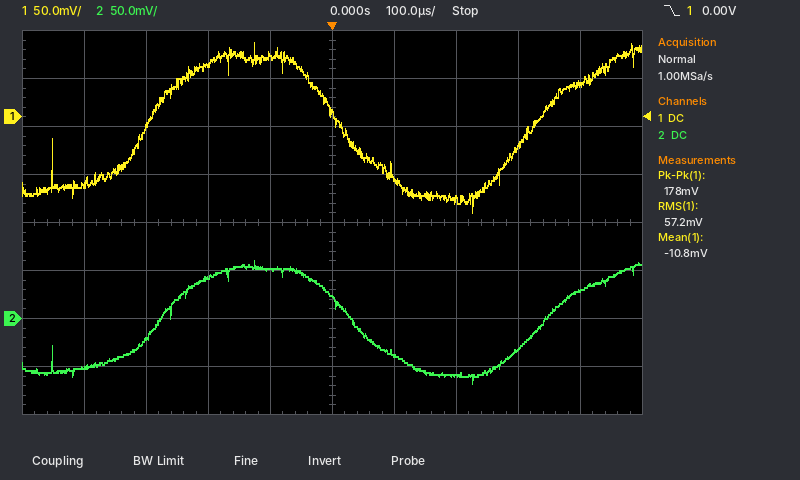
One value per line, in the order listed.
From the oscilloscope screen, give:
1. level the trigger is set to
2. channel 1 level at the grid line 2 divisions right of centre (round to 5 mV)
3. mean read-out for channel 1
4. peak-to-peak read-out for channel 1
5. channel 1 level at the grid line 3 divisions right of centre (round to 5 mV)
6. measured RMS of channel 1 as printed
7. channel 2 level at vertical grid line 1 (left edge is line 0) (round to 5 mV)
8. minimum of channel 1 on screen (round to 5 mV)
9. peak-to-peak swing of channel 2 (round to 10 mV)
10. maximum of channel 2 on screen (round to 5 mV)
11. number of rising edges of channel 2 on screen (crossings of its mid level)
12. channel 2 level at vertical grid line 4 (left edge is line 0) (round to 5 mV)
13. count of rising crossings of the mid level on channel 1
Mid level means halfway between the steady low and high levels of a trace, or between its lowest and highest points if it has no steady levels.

0.00 V
-85 mV
-10.8 mV
178 mV
-30 mV
57.2 mV
-50 mV
-100 mV
130 mV
60 mV
2
50 mV
2
